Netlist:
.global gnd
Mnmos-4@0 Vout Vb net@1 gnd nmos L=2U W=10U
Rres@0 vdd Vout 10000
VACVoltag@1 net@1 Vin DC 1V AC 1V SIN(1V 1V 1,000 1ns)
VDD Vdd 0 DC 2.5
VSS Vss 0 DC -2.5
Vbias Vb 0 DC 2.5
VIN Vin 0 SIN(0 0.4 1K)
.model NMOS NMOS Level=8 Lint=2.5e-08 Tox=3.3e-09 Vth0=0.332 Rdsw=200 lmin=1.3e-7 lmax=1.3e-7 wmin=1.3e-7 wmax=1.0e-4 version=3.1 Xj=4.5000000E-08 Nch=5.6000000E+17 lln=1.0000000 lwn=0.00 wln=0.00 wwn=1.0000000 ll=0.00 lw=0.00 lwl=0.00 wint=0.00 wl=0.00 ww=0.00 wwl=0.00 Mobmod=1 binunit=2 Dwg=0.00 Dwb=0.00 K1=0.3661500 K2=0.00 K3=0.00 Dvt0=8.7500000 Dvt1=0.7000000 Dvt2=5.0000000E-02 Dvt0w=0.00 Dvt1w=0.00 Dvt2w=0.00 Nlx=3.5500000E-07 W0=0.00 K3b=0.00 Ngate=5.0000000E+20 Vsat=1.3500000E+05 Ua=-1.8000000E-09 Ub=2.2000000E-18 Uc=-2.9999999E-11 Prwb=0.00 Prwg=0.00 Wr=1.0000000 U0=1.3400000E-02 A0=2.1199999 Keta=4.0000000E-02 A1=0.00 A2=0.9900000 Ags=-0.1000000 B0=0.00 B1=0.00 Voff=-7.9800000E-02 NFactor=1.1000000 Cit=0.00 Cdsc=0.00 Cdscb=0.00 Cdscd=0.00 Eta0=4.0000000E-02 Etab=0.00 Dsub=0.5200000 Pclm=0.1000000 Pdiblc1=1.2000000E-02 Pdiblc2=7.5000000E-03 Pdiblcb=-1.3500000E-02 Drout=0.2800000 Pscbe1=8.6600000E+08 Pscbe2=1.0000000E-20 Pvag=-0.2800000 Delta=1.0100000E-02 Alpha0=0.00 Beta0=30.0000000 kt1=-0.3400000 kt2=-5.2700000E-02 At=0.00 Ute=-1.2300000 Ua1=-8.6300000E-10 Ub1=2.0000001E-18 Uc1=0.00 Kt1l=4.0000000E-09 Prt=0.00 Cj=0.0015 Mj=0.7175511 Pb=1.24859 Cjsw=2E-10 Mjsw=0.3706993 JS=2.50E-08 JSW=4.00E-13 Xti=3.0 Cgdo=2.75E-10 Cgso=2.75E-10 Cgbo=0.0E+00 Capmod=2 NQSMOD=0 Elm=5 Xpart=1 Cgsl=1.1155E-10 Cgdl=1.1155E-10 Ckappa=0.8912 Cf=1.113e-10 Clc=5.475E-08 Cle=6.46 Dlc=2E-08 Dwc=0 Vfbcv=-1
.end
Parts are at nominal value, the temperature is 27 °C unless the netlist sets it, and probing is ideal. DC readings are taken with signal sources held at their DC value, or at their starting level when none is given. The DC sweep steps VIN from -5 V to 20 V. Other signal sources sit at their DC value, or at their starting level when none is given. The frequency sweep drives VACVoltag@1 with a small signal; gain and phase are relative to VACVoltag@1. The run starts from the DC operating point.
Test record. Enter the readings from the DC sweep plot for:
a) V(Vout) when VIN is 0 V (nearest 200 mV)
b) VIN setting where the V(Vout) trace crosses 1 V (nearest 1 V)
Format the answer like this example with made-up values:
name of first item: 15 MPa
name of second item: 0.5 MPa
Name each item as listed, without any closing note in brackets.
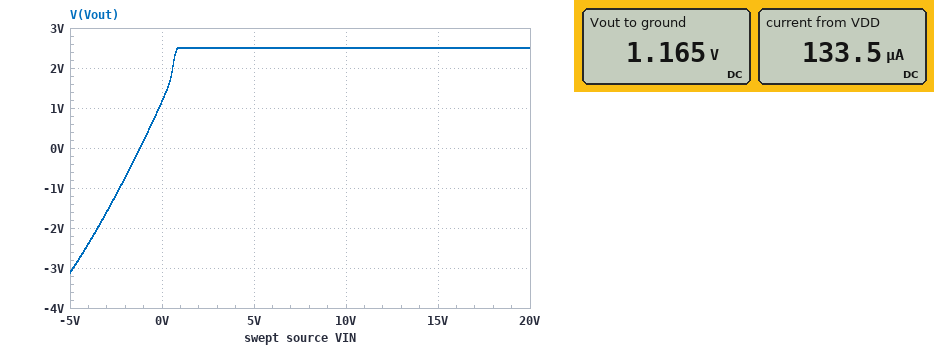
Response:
V(Vout) when VIN is 0 V: 1.2 V
VIN setting where the V(Vout) trace crosses 1 V: 0 V
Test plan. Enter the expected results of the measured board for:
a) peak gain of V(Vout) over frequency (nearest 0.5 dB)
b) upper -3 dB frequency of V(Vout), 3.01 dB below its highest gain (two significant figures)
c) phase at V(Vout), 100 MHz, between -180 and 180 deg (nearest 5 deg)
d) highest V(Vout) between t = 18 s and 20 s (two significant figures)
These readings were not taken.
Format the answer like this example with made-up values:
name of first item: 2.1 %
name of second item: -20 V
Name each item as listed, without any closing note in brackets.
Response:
peak gain of V(Vout) over frequency: 0.5 dB
upper -3 dB frequency of V(Vout), 3.01 dB below its highest gain: 800 MHz
phase at V(Vout), 100 MHz, between -180 and 180 deg: -5 deg
highest V(Vout) between t = 18 s and 20 s: 2.5 V
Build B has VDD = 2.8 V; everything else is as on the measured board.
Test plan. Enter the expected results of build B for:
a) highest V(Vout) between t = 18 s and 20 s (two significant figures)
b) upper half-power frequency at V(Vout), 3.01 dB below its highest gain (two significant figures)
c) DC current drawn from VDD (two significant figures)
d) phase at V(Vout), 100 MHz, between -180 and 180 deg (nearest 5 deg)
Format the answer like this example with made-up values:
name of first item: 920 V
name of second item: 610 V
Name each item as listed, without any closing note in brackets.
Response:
highest V(Vout) between t = 18 s and 20 s: 2.8 V
upper half-power frequency at V(Vout), 3.01 dB below its highest gain: 760 MHz
DC current drawn from VDD: 160 µA
phase at V(Vout), 100 MHz, between -180 and 180 deg: -5 deg
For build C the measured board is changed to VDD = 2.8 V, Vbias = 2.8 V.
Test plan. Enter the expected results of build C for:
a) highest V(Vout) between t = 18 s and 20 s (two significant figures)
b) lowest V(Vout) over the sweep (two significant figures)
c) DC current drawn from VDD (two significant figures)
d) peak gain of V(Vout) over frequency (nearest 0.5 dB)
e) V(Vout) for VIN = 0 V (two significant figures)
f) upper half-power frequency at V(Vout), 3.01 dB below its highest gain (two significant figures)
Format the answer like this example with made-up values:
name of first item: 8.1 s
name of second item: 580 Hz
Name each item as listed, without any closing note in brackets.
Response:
highest V(Vout) between t = 18 s and 20 s: 2.8 V
lowest V(Vout) over the sweep: -3.0 V
DC current drawn from VDD: 160 µA
peak gain of V(Vout) over frequency: 0 dB
V(Vout) for VIN = 0 V: 1.2 V
upper half-power frequency at V(Vout), 3.01 dB below its highest gain: 950 MHz
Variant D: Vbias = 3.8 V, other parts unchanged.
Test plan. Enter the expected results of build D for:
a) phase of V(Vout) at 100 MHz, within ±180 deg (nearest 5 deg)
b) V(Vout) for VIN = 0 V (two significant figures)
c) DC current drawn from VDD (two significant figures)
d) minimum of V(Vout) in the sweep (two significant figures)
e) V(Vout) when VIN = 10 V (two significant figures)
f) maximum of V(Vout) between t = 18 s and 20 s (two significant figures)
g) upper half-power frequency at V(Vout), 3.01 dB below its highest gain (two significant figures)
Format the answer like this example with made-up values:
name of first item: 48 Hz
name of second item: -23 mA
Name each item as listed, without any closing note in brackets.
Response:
phase of V(Vout) at 100 MHz, within ±180 deg: -5 deg
V(Vout) for VIN = 0 V: 1.1 V
DC current drawn from VDD: 140 µA
minimum of V(Vout) in the sweep: -2.9 V
V(Vout) when VIN = 10 V: 2.8 V
maximum of V(Vout) between t = 18 s and 20 s: 2.4 V
upper half-power frequency at V(Vout), 3.01 dB below its highest gain: 1.1 GHz
